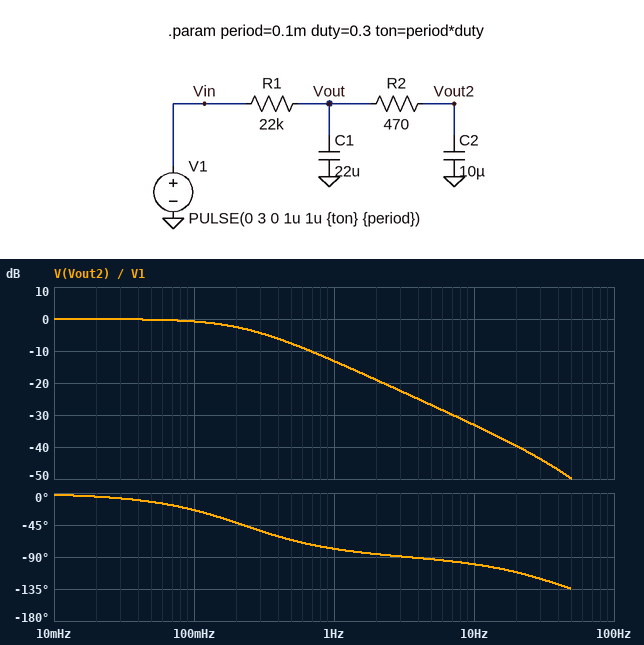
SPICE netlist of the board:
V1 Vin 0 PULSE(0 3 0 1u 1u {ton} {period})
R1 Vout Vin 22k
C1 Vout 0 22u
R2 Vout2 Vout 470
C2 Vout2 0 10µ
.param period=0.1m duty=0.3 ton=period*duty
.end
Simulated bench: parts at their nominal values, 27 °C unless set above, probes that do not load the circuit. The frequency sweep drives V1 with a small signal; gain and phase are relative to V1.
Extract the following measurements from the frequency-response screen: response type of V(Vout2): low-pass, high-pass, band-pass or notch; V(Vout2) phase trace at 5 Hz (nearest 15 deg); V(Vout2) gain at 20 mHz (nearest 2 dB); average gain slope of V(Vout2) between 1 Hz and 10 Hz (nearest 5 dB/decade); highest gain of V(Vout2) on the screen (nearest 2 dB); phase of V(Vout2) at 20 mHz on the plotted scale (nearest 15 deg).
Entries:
low-pass
-90 deg
0 dB
-20 dB/decade
0 dB
0 deg
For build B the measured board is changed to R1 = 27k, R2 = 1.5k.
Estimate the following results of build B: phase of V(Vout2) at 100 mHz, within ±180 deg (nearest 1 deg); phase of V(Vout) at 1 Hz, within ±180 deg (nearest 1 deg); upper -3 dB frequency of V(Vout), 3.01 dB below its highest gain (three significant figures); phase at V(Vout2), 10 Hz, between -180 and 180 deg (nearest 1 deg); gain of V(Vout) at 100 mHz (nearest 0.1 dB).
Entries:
-29 deg
-78 deg
183 mHz
-122 deg
-1.1 dB
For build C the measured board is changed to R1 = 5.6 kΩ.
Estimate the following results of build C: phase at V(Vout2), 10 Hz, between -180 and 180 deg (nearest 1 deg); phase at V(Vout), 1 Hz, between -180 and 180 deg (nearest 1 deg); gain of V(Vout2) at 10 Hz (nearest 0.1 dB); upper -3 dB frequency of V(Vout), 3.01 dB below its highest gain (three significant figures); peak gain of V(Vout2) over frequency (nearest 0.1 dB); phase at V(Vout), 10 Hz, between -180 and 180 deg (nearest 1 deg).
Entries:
-96 deg
-48 deg
-21.3 dB
881 mHz
0 dB
-80 deg
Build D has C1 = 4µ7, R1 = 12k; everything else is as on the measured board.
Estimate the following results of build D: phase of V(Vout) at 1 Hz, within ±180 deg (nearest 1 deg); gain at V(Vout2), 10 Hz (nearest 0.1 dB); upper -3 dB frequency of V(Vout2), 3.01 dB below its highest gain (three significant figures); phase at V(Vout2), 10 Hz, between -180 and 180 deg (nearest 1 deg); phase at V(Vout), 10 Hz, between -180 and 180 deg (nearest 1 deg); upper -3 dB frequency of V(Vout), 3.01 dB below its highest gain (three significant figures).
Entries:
-47 deg
-21.1 dB
886 mHz
-90 deg
-74 deg
887 mHz
